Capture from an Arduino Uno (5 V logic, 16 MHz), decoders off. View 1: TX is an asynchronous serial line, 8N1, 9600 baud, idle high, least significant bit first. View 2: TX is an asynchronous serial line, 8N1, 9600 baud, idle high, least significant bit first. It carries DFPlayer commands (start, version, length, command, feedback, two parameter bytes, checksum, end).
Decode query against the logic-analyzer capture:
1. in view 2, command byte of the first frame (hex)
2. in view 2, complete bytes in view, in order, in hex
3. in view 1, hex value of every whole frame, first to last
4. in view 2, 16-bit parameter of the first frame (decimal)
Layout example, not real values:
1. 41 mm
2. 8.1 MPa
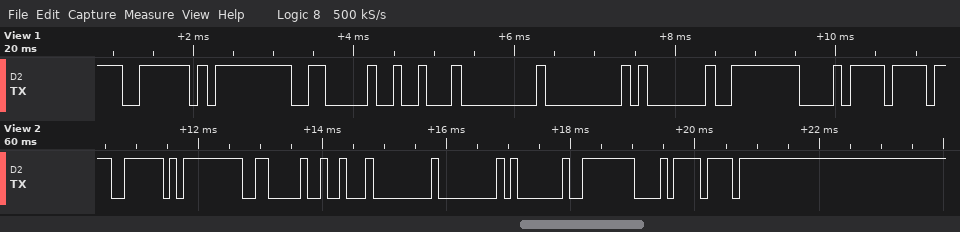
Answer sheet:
1. 0x12
2. 0x7E 0xFF 0x06 0x12 0x00 0x00 0x01 0xFE 0xE8 0xEF
3. 7E FF 06 12 00 00 01 FE E8
4. 1
